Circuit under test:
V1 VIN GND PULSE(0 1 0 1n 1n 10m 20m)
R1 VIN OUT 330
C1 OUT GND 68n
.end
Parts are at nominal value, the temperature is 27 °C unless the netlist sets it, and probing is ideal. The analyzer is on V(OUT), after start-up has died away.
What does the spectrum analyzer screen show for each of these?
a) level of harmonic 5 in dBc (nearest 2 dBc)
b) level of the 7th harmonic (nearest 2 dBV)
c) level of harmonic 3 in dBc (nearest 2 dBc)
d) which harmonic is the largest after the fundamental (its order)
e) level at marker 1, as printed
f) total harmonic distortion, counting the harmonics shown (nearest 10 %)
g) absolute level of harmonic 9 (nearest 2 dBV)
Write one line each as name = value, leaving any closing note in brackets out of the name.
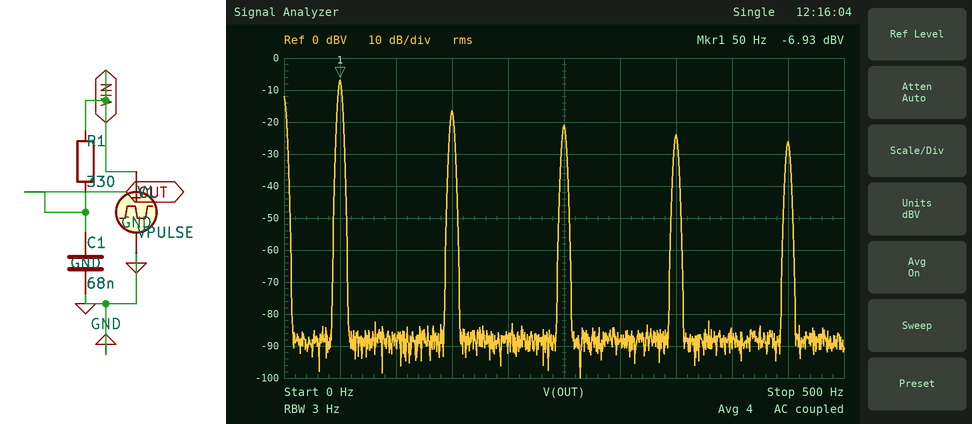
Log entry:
level of harmonic 5 in dBc = -14 dBc
level of the 7th harmonic = -24 dBV
level of harmonic 3 in dBc = -10 dBc
which harmonic is the largest after the fundamental = 3
level at marker 1, as printed = -6.93 dBV
total harmonic distortion, counting the harmonics shown = 40 %
absolute level of harmonic 9 = -26 dBV
